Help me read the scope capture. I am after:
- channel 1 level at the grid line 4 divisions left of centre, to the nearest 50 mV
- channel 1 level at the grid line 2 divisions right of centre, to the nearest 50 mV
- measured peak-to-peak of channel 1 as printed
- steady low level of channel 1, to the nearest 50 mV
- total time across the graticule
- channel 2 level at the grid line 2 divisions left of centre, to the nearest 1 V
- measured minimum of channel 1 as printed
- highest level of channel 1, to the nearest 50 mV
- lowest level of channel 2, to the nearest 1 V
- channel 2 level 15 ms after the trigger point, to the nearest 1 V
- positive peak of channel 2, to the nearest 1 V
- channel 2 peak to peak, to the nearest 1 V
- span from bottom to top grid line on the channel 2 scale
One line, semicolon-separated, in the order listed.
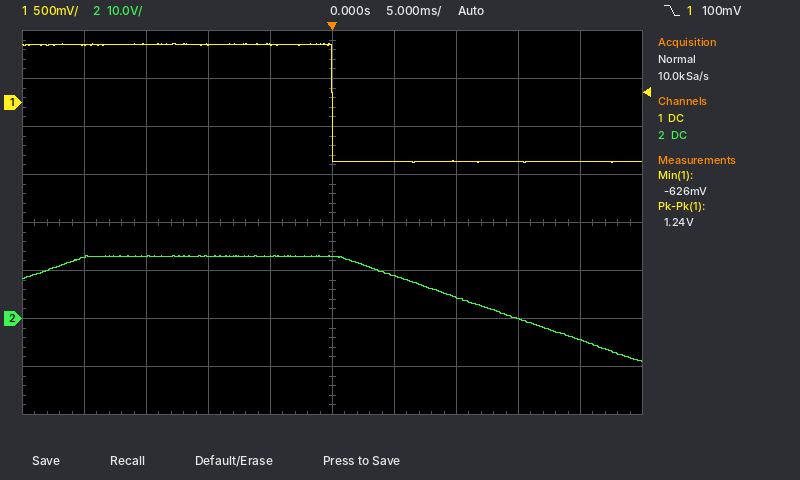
600 mV; -600 mV; 1.24 V; -600 mV; 50 ms; 13 V; -626 mV; 600 mV; -9 V; 0 V; 13 V; 22 V; 80 V
